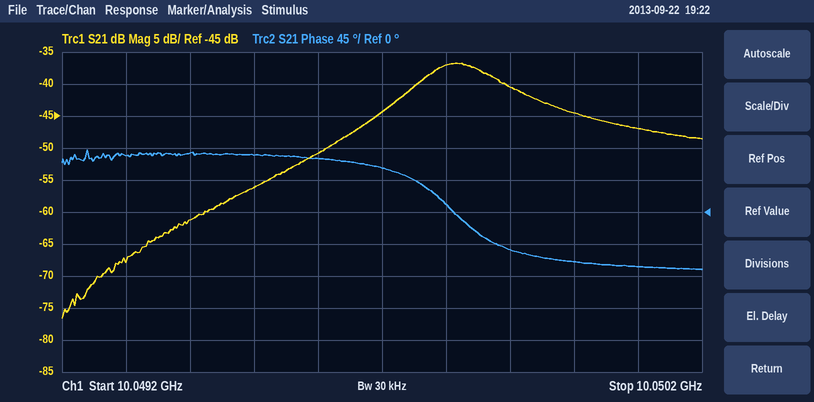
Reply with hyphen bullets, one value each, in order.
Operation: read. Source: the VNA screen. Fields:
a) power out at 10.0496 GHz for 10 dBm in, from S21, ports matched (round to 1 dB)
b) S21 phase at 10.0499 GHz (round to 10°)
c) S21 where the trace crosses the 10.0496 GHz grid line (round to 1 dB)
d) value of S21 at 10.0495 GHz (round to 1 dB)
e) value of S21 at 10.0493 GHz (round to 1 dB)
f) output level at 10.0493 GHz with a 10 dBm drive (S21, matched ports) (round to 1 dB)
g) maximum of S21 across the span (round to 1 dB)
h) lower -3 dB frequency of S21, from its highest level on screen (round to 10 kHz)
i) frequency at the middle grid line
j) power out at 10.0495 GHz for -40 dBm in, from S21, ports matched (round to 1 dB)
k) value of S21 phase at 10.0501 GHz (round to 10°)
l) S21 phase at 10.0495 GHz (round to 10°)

- -41 dBm
- -50°
- -51 dB
- -56 dB
- -68 dB
- -58 dBm
- -37 dB
- 10.04976 GHz
- 10.0497 GHz
- -96 dBm
- -80°
- 80°
